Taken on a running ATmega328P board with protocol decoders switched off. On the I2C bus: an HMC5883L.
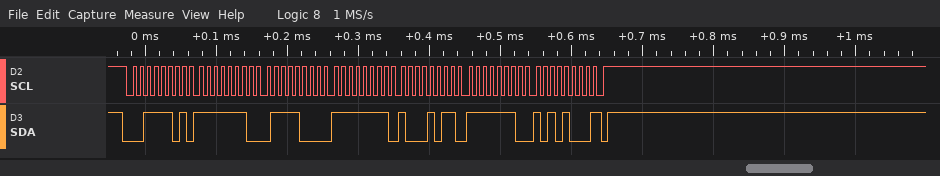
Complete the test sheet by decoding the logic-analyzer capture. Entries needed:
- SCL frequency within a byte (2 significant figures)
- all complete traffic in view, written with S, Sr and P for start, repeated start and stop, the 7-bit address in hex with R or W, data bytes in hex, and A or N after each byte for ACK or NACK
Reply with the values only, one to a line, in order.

100 kHz
S 1ER A FE A 78 A FF A 8B A FE A A8 N P
